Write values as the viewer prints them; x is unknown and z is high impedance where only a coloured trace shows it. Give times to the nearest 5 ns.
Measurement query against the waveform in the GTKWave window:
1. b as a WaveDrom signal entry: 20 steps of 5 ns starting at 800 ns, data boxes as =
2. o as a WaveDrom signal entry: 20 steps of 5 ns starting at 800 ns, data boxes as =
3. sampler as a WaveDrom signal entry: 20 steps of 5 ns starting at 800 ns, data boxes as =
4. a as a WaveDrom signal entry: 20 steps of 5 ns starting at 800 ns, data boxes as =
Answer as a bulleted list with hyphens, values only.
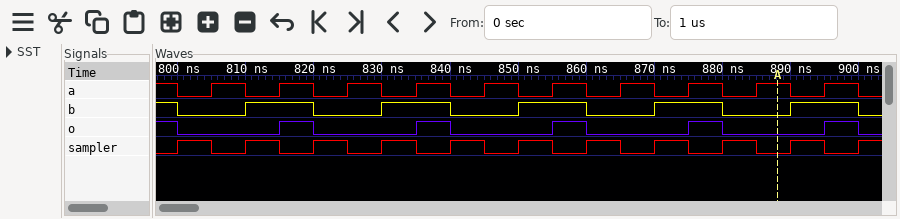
- {name: 'b', wave: '0.1.0.1.0.1.0.1.0.1.'}
- {name: 'o', wave: '0..10..10..10..10..1'}
- {name: 'sampler', wave: '10101010101010101010'}
- {name: 'a', wave: '01010101010101010101'}
